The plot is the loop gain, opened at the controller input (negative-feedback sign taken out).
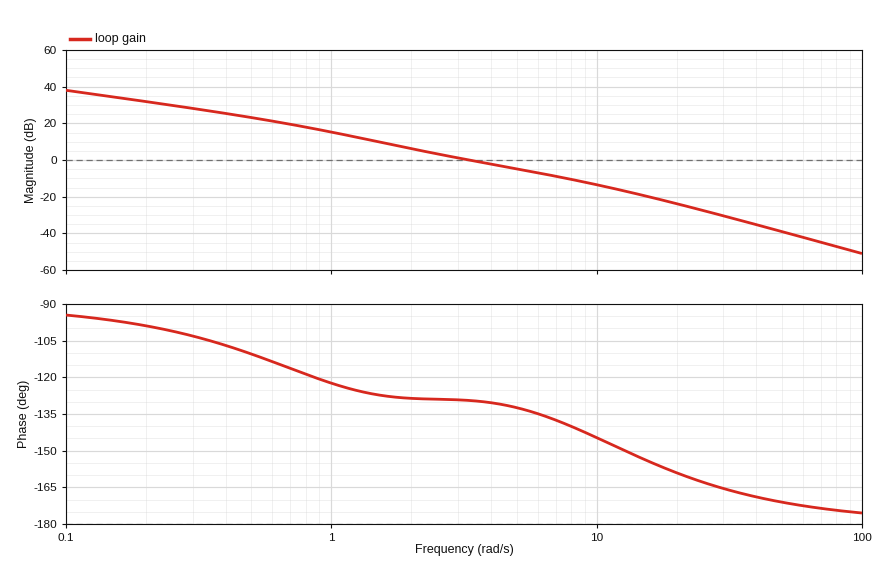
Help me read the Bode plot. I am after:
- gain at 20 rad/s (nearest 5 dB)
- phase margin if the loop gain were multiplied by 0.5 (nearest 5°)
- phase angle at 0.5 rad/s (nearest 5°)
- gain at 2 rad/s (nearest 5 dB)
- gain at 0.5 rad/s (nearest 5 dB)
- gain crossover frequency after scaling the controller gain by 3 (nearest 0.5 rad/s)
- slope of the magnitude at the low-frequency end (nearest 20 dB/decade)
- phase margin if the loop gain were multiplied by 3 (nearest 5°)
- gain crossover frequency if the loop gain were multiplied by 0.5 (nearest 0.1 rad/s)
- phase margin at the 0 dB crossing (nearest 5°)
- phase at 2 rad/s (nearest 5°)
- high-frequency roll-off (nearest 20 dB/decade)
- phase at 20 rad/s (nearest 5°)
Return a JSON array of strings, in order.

["-25 dB", "50°", "-110°", "5 dB", "25 dB", "7.5 rad/s", "-20 dB/decade", "40°", "2.0 rad/s", "50°", "-130°", "-40 dB/decade", "-160°"]
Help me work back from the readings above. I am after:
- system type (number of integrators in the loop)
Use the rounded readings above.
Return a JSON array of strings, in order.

["1"]
